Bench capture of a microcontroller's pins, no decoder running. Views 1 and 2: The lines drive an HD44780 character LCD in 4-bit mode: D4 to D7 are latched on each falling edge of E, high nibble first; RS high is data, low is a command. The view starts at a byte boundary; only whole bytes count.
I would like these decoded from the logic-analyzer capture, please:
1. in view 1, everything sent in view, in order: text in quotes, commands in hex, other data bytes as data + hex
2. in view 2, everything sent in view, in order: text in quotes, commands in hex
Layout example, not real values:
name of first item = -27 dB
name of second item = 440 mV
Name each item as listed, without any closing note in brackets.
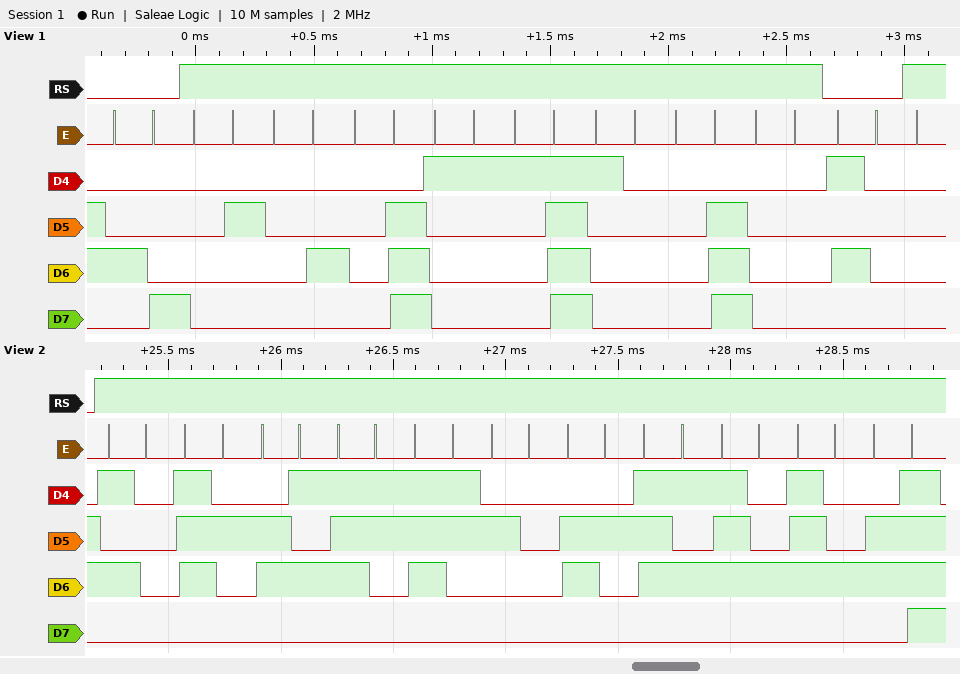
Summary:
in view 1, everything sent in view, in order: text in quotes, commands in hex, other data bytes as data + hex = 0x48 data 02 04 0E 11 1F 10 0E 00 0x50
in view 2, everything sent in view, in order: text in quotes, commands in hex = "Press butto"
